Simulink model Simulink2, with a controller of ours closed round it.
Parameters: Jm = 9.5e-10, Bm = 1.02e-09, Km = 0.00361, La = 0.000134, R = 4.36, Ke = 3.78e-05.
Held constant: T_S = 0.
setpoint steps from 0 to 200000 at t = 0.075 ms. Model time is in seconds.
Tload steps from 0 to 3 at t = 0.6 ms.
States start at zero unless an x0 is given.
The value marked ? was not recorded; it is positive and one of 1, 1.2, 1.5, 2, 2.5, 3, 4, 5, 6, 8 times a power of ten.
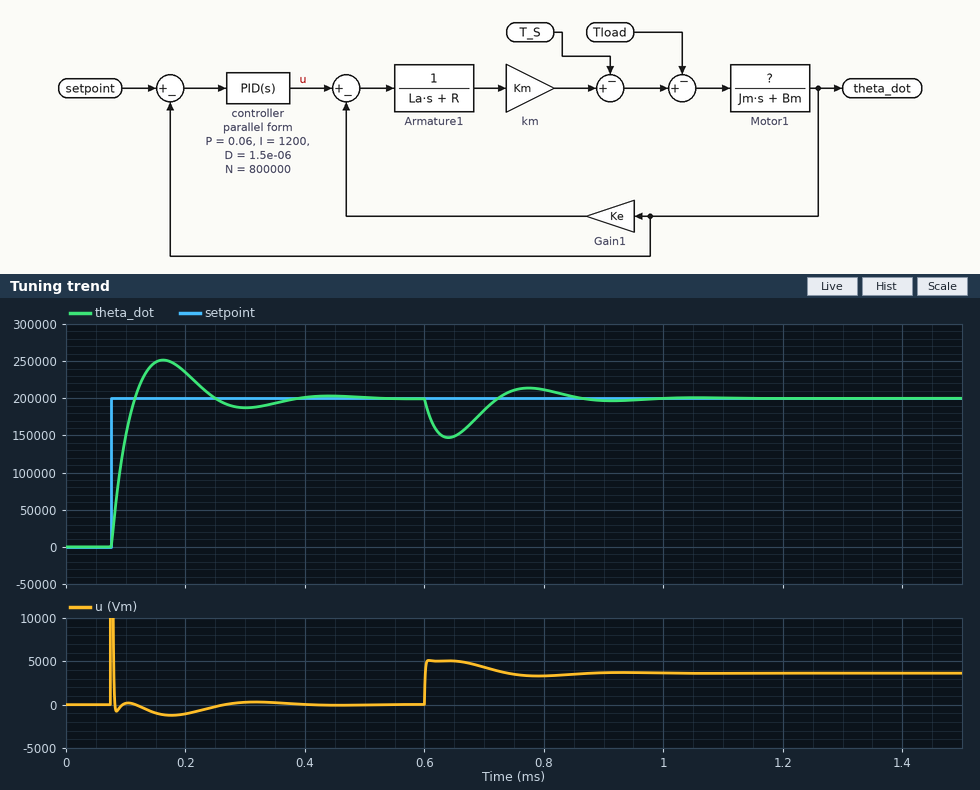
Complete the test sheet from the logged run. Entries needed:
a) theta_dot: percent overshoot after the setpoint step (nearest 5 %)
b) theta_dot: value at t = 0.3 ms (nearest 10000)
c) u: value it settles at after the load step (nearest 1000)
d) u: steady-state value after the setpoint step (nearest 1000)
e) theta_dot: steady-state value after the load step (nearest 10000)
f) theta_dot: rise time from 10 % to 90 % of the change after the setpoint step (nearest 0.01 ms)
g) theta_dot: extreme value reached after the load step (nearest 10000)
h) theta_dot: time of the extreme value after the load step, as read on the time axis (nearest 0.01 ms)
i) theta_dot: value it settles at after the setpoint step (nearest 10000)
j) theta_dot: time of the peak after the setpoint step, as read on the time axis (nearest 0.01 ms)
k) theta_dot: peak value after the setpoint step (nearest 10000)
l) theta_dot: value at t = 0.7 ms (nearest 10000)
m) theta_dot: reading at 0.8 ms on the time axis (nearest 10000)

25 %
190000
4000
0
200000
0.03 ms
150000
0.64 ms
200000
0.16 ms
250000
180000
210000
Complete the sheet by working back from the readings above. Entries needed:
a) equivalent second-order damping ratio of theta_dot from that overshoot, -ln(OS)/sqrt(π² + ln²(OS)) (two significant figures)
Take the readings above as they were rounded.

0.40
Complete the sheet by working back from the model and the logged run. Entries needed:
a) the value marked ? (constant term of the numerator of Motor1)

1
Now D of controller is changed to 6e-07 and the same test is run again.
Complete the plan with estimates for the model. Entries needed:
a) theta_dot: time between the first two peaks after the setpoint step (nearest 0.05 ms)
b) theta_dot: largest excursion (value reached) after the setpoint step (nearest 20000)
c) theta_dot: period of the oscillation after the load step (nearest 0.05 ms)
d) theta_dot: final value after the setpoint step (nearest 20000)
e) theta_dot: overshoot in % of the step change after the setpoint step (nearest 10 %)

0.20 ms
300000
0.20 ms
200000
50 %
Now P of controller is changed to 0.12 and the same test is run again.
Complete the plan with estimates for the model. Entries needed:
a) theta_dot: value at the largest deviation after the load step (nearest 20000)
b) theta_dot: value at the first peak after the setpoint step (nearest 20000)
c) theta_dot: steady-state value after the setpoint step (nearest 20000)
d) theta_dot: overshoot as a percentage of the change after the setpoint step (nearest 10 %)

160000
240000
200000
20 %
